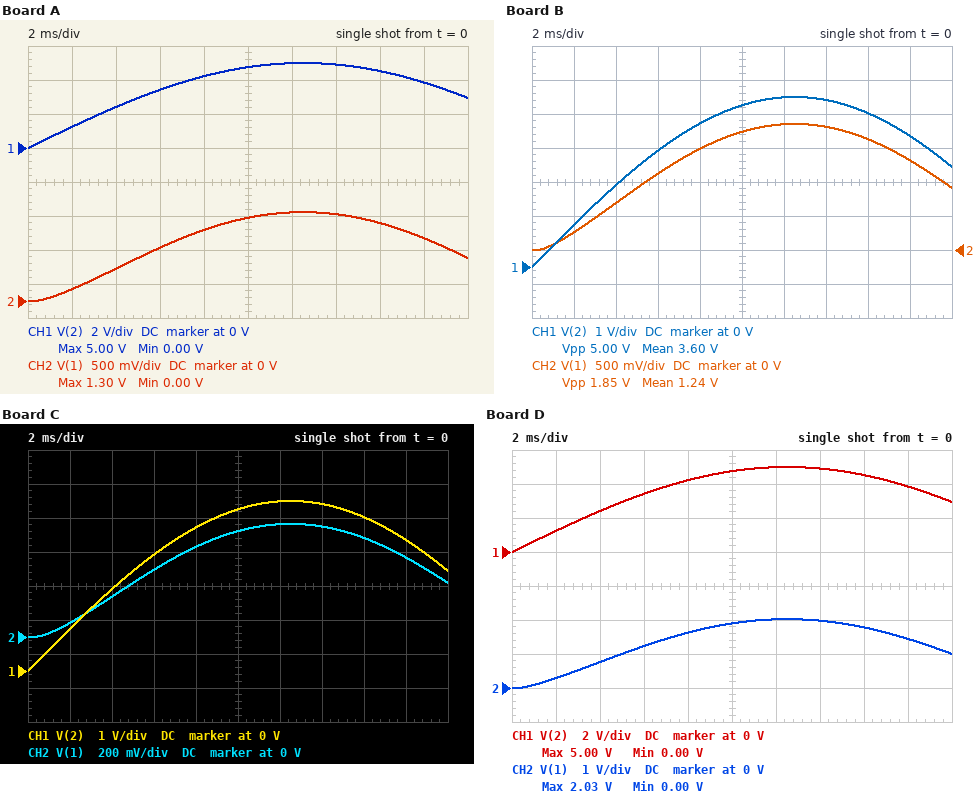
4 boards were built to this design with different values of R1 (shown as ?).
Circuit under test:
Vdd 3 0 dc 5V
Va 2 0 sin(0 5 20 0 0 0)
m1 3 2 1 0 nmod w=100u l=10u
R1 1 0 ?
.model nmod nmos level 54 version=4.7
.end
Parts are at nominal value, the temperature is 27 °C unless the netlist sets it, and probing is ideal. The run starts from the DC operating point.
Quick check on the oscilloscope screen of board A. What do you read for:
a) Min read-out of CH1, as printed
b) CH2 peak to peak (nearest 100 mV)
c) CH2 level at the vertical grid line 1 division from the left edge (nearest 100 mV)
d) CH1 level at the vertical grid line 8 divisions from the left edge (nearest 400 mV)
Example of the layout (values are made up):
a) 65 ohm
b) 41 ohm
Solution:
a) 0.00 V
b) 1.3 V
c) 200 mV
d) 4.4 V
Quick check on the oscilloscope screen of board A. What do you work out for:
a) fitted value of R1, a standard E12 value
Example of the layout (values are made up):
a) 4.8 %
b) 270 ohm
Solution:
a) 82 Ω
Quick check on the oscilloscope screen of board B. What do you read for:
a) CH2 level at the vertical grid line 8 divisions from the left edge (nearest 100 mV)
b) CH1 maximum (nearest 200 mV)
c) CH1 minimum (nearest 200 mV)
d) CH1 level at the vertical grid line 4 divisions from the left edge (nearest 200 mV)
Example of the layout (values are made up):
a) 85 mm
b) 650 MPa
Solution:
a) 1.6 V
b) 5.0 V
c) 0 V
d) 4.2 V
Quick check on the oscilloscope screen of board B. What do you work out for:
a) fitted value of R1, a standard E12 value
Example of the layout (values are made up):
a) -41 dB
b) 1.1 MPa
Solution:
a) 150 Ω
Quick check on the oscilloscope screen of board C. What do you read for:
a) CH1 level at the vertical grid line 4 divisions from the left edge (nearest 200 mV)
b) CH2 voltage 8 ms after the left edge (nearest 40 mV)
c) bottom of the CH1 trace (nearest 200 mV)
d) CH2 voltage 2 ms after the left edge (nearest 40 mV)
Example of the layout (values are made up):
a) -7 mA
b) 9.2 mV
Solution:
a) 4.2 V
b) 520 mV
c) 0 V
d) 80 mV
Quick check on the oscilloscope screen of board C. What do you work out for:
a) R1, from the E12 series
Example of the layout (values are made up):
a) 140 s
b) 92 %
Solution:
a) 33 Ω
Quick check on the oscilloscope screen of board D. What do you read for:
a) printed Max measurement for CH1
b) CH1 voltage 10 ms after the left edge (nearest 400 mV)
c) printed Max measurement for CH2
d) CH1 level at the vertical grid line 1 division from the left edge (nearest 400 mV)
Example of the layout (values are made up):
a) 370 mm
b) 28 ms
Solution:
a) 5.00 V
b) 4.8 V
c) 2.03 V
d) 1.2 V
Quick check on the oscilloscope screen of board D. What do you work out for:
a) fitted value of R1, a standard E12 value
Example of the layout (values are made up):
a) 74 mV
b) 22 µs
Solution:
a) 180 Ω
